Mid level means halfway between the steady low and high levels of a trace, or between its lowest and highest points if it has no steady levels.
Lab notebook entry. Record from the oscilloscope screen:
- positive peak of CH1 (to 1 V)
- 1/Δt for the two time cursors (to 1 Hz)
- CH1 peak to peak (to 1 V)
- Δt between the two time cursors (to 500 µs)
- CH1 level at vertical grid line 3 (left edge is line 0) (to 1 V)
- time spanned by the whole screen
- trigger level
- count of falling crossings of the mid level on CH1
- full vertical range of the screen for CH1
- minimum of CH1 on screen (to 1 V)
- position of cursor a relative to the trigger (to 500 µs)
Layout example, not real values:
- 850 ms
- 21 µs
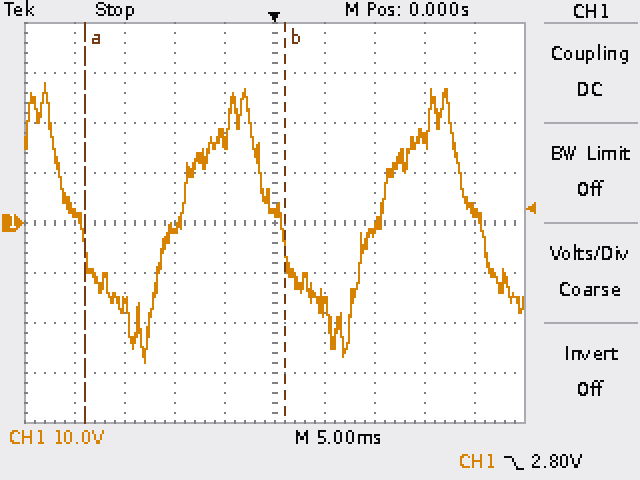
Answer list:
- 28 V
- 50 Hz
- 56 V
- 20.0 ms
- -1 V
- 50 ms
- 2.80 V
- 3
- 80 V
- -28 V
- -19.0 ms
